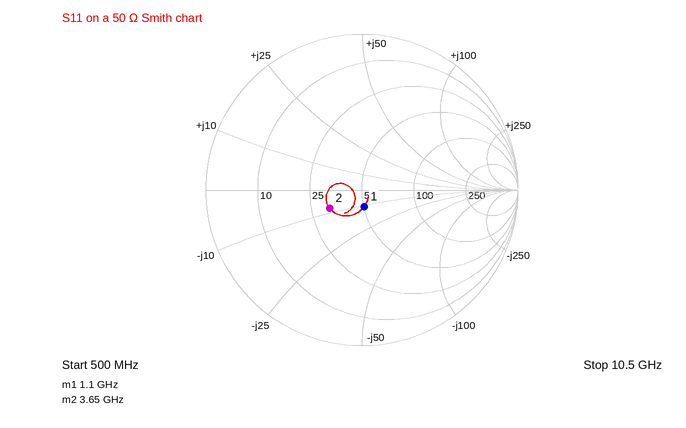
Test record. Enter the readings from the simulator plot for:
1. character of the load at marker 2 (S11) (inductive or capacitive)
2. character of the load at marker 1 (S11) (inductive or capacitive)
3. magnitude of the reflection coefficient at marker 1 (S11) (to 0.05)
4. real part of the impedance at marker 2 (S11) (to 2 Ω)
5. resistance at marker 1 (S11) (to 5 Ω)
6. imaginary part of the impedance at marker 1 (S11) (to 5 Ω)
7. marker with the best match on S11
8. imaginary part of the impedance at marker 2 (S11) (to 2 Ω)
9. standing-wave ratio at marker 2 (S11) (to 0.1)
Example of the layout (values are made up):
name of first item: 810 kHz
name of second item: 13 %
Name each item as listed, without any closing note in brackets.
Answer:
character of the load at marker 2 (S11): capacitive
character of the load at marker 1 (S11): capacitive
magnitude of the reflection coefficient at marker 1 (S11): 0.10
real part of the impedance at marker 2 (S11): 32 Ω
resistance at marker 1 (S11): 50 Ω
imaginary part of the impedance at marker 1 (S11): -10 Ω
marker with the best match on S11: marker 1
imaginary part of the impedance at marker 2 (S11): -8 Ω
standing-wave ratio at marker 2 (S11): 1.6
